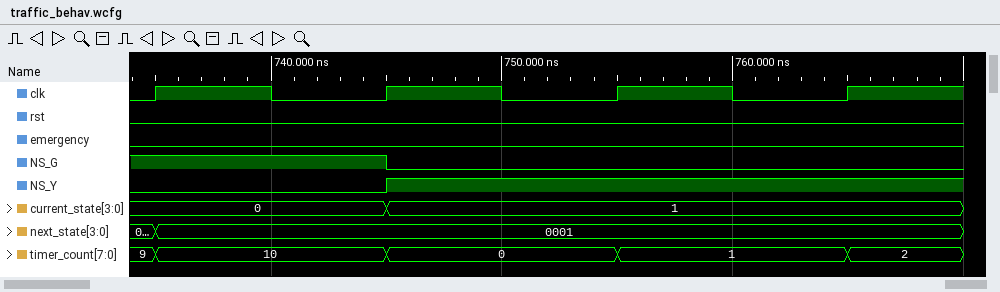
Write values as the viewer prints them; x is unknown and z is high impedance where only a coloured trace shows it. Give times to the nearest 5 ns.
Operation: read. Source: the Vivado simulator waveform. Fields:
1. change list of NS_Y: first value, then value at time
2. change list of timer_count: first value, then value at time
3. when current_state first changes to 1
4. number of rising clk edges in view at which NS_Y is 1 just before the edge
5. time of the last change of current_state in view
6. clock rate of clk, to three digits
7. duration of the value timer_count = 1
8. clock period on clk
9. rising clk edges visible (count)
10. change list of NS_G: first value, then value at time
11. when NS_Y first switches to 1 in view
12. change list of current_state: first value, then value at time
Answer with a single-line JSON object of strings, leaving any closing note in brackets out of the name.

{"change list of NS_Y: first value, then value at time": "0, 1 at 745 ns", "change list of timer_count: first value, then value at time": "9, 10 at 735 ns, 0 at 745 ns, 1 at 755 ns, 2 at 765 ns", "when current_state first changes to 1": "745 ns", "number of rising clk edges in view at which NS_Y is 1 just before the edge": "2", "time of the last change of current_state in view": "745 ns", "clock rate of clk, to three digits": "100 MHz", "duration of the value timer_count = 1": "10 ns", "clock period on clk": "10 ns", "rising clk edges visible": "4", "change list of NS_G: first value, then value at time": "1, 0 at 745 ns", "when NS_Y first switches to 1 in view": "745 ns", "change list of current_state: first value, then value at time": "0, 1 at 745 ns"}
